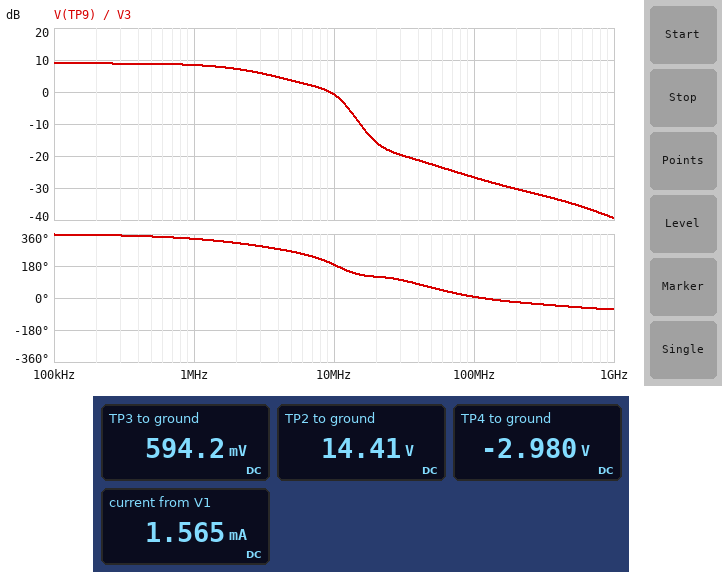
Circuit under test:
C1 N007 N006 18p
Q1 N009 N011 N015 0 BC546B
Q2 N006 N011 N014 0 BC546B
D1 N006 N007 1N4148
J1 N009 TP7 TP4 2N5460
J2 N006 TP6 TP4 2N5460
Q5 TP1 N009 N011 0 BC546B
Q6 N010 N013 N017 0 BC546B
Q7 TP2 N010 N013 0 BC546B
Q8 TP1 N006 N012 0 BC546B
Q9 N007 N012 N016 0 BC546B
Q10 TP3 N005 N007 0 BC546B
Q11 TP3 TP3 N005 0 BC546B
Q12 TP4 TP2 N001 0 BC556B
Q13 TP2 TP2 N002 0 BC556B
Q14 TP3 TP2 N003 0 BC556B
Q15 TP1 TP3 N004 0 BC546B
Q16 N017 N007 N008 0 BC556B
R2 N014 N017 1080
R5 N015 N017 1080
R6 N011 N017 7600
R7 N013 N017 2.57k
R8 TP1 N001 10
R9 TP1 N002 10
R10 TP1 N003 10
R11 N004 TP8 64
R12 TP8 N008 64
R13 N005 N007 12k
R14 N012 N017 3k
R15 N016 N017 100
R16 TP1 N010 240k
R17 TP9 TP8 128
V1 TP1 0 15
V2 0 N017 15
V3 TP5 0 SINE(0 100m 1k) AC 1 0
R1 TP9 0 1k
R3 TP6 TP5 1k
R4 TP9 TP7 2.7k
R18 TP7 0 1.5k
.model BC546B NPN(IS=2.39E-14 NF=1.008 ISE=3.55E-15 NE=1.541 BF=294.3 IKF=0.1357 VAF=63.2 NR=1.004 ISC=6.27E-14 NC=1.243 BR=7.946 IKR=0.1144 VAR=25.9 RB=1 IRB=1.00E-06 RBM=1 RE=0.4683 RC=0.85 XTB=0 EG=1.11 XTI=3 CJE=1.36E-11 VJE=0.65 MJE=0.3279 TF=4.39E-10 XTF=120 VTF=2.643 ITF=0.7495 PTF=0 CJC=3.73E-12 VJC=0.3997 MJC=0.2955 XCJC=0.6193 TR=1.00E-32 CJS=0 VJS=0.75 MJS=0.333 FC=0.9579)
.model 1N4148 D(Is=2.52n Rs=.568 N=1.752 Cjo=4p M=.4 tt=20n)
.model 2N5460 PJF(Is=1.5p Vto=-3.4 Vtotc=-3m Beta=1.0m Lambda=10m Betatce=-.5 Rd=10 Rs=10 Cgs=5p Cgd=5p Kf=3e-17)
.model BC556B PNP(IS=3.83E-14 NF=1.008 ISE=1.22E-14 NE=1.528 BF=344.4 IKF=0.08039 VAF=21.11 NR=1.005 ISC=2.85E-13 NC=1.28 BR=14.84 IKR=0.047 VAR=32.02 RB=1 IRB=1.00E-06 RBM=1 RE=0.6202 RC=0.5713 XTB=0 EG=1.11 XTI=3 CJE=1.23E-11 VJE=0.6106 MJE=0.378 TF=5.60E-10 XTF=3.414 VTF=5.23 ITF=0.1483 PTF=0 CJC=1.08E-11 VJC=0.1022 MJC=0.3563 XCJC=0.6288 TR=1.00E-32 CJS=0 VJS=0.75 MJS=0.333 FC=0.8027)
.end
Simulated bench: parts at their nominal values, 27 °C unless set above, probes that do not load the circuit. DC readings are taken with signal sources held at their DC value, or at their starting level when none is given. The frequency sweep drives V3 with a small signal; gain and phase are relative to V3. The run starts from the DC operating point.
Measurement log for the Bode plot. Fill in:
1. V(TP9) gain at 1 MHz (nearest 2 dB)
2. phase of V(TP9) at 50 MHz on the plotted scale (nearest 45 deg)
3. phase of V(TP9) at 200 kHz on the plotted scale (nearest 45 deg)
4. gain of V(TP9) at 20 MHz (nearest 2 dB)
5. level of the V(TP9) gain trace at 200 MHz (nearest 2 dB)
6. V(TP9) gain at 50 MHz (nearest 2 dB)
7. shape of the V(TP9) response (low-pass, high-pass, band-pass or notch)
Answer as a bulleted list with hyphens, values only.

- 8 dB
- 45 deg
- 360 deg
- -16 dB
- -30 dB
- -22 dB
- low-pass
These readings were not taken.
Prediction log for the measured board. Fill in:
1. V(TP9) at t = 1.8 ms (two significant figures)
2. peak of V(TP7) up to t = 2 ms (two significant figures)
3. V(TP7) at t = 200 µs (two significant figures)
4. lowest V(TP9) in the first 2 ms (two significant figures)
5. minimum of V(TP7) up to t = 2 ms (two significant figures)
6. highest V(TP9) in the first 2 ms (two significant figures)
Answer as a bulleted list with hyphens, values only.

- -270 mV
- 100 mV
- 95 mV
- -280 mV
- -100 mV
- 280 mV
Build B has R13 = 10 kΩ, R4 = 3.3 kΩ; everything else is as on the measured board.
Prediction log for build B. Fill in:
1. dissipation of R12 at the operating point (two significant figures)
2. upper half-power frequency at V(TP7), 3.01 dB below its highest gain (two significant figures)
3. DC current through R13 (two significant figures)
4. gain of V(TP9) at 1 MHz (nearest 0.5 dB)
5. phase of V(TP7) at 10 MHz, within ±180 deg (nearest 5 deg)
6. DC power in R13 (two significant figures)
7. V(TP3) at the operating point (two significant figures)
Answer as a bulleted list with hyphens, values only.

- 1.7 µW
- 2.3 MHz
- 61 µA
- 9.5 dB
- 140 deg
- 37 µW
- 600 mV
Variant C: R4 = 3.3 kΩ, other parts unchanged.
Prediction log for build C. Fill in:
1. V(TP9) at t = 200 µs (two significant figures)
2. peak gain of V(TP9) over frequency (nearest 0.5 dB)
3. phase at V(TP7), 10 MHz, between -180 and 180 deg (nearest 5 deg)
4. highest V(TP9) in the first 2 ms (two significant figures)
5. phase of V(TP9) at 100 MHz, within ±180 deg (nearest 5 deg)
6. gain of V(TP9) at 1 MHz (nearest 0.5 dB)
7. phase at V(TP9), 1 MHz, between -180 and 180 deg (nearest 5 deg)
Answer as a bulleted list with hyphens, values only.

- 300 mV
- 10.0 dB
- 140 deg
- 320 mV
- 10 deg
- 9.5 dB
- -30 deg
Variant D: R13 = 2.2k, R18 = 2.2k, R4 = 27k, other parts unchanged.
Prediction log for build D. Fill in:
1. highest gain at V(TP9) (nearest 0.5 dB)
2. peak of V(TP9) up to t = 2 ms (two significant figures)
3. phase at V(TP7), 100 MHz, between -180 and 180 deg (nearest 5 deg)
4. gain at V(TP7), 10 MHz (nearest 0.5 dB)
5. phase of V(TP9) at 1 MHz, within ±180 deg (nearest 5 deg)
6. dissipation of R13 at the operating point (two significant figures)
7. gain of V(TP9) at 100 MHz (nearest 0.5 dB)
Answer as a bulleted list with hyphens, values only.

- 22.5 dB
- 1.3 V
- -45 deg
- -12.0 dB
- -70 deg
- 150 µW
- -27.0 dB
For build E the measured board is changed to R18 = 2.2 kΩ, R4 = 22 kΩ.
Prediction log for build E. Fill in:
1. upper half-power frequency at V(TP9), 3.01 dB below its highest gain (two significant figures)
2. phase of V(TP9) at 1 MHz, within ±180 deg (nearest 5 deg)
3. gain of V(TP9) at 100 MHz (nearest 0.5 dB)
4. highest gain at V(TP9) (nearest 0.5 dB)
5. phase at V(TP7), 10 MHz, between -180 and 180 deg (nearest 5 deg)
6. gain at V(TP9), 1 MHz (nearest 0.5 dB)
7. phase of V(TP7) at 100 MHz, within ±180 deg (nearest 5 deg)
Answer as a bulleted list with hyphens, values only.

- 590 kHz
- -65 deg
- -27.0 dB
- 21.0 dB
- 60 deg
- 15.0 dB
- -45 deg
